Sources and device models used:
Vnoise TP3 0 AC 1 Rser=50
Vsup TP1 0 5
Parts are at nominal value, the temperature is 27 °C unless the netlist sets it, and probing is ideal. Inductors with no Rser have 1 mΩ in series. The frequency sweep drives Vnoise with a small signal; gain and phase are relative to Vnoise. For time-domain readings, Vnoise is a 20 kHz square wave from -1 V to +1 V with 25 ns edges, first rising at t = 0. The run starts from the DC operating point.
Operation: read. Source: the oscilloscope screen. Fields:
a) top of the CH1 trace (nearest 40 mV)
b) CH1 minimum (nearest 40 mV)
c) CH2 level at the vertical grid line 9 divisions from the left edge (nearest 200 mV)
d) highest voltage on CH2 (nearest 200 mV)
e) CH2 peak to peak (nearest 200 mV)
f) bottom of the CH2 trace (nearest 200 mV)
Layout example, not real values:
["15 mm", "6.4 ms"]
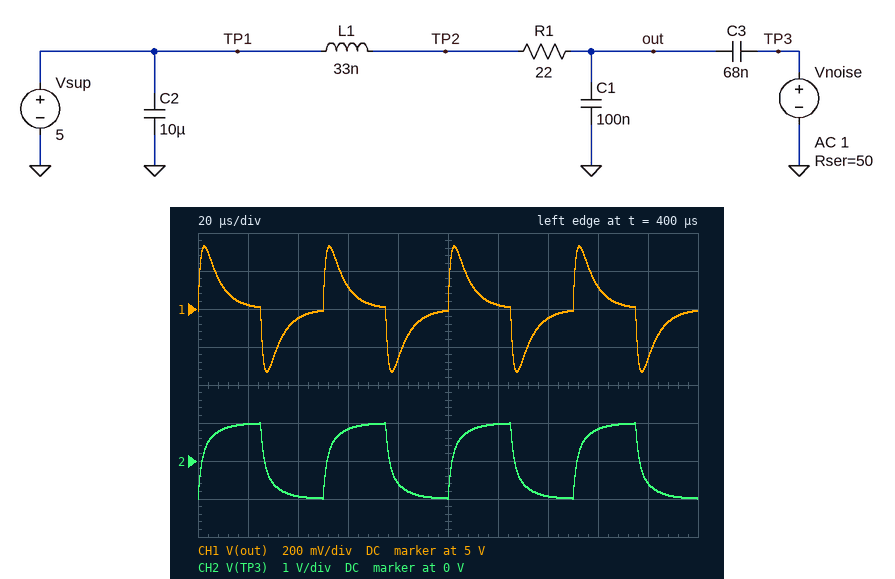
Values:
["5.32 V", "4.68 V", "-600 mV", "1.0 V", "2.0 V", "-1.0 V"]
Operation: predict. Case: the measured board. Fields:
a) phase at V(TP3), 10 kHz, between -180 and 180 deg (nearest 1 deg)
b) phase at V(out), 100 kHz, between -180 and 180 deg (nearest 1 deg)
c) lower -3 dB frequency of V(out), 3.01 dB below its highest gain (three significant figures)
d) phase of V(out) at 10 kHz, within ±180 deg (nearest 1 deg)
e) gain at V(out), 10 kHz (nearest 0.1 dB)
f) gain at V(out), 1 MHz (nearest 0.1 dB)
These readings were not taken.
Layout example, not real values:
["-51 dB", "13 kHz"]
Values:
["-12 deg", "-24 deg", "19.8 kHz", "65 deg", "-21.1 dB", "-30.0 dB"]
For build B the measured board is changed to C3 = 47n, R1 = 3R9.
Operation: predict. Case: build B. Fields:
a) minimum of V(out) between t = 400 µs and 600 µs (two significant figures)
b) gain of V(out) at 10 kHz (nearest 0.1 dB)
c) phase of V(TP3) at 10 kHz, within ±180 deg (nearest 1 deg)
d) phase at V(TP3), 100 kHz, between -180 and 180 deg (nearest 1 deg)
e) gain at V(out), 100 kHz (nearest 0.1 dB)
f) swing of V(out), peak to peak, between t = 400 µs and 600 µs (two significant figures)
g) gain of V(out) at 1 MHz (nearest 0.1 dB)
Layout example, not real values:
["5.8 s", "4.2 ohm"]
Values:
["4.9 V", "-38.9 dB", "-8 deg", "-51 deg", "-24.5 dB", "210 mV", "-30.6 dB"]
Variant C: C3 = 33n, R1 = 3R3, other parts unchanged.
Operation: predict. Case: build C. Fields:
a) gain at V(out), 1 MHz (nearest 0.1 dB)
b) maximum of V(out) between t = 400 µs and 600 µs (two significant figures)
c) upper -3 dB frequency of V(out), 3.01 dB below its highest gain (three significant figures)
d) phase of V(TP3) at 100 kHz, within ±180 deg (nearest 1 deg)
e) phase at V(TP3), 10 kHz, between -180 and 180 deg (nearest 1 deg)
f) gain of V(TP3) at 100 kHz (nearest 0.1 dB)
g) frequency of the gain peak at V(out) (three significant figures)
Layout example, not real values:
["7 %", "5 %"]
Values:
["-30.8 dB", "5.1 V", "696 kHz", "-44 deg", "-6 deg", "-3.4 dB", "219 kHz"]
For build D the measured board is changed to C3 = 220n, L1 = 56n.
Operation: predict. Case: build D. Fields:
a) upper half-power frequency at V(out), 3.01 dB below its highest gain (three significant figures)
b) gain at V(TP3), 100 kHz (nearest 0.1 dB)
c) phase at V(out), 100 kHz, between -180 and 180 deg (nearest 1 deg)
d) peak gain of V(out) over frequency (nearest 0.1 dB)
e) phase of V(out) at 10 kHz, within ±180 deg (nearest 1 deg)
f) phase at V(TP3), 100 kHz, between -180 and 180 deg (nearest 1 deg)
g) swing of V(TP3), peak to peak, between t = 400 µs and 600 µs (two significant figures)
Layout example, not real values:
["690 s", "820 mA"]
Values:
["127 kHz", "-9.9 dB", "-37 deg", "-11.4 dB", "39 deg", "-50 deg", "1.5 V"]
